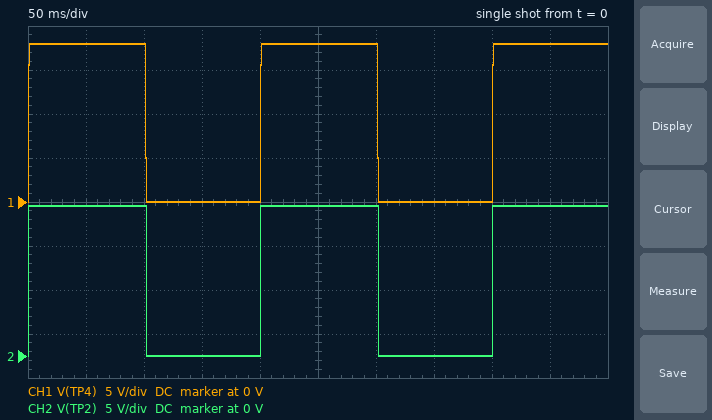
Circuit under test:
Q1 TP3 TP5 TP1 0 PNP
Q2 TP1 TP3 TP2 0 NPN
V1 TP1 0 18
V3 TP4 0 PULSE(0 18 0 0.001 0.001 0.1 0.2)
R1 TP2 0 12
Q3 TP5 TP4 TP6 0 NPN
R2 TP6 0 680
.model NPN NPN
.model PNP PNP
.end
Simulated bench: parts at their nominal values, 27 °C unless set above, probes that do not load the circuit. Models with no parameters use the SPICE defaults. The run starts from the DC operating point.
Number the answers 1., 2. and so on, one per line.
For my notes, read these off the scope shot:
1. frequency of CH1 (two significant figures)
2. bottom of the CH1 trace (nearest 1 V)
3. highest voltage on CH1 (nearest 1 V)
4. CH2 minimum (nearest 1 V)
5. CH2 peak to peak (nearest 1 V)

1. 5.0 Hz
2. 0 V
3. 18 V
4. 0 V
5. 17 V
